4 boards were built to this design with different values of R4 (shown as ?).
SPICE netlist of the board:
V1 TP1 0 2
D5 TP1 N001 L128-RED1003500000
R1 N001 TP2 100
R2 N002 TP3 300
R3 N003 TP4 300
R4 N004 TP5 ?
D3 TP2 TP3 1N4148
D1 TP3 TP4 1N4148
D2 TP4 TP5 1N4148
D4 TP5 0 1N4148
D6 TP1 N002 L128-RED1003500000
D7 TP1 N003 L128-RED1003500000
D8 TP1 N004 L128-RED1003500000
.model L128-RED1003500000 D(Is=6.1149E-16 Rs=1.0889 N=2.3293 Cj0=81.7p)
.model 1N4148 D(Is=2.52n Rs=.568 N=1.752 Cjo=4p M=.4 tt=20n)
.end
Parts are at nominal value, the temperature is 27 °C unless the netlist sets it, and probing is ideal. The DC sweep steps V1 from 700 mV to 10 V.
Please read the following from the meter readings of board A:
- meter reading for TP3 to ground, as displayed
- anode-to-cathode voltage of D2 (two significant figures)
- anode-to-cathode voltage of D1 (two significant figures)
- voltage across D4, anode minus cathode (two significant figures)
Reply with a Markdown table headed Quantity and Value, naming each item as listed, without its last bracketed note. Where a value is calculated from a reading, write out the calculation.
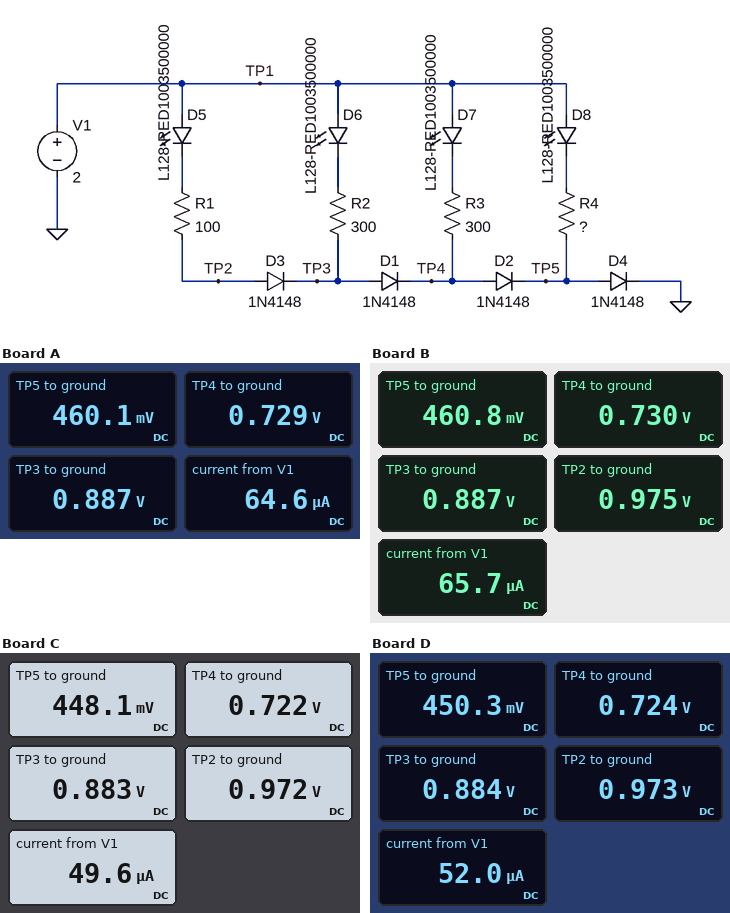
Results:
| Quantity | Value |
|---|---|
| meter reading for TP3 to ground, as displayed | 0.887 V |
| anode-to-cathode voltage of D2 | 729 mV - 460.1 mV = 270 mV |
| anode-to-cathode voltage of D1 | 887 mV - 729 mV = 160 mV |
| voltage across D4, anode minus cathode | 460.1 mV = 460 mV |
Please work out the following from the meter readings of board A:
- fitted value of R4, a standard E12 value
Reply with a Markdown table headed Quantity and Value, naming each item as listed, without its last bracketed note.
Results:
| Quantity | Value |
|---|---|
| fitted value of R4, a standard E12 value | 180 Ω |
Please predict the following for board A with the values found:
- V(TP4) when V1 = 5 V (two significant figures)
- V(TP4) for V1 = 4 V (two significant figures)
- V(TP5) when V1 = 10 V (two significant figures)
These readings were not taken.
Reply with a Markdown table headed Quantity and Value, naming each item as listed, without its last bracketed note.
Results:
| Quantity | Value |
|---|---|
| V(TP4) when V1 = 5 V | 1.5 V |
| V(TP4) for V1 = 4 V | 1.4 V |
| V(TP5) when V1 = 10 V | 880 mV |
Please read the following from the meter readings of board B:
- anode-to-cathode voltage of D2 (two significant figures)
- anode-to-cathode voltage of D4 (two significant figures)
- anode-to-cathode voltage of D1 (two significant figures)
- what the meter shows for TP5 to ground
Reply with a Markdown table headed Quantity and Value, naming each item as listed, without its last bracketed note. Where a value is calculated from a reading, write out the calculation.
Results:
| Quantity | Value |
|---|---|
| anode-to-cathode voltage of D2 | 730 mV - 460.8 mV = 270 mV |
| anode-to-cathode voltage of D4 | 460.8 mV = 460 mV |
| anode-to-cathode voltage of D1 | 887 mV - 730 mV = 160 mV |
| what the meter shows for TP5 to ground | 460.8 mV |
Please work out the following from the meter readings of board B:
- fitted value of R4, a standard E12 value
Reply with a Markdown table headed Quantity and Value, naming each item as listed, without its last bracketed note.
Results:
| Quantity | Value |
|---|---|
| fitted value of R4, a standard E12 value | 150 Ω |
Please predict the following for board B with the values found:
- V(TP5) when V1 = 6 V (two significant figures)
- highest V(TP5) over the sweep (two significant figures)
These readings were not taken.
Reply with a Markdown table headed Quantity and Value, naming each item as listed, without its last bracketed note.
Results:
| Quantity | Value |
|---|---|
| V(TP5) when V1 = 6 V | 790 mV |
| highest V(TP5) over the sweep | 880 mV |
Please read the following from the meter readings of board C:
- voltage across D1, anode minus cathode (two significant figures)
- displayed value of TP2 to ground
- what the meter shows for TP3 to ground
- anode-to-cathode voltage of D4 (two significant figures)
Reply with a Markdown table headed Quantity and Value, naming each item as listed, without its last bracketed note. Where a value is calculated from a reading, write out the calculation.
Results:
| Quantity | Value |
|---|---|
| voltage across D1, anode minus cathode | 883 mV - 722 mV = 160 mV |
| displayed value of TP2 to ground | 0.972 V |
| what the meter shows for TP3 to ground | 0.883 V |
| anode-to-cathode voltage of D4 | 448.1 mV = 450 mV |
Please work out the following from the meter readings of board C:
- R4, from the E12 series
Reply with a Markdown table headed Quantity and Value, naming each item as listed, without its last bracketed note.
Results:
| Quantity | Value |
|---|---|
| R4, from the E12 series | 820 Ω |
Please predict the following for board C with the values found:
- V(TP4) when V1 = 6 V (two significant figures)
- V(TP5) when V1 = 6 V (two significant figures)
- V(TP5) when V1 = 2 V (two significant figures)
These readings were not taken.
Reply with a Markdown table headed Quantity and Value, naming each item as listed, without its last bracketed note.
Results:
| Quantity | Value |
|---|---|
| V(TP4) when V1 = 6 V | 1.5 V |
| V(TP5) when V1 = 6 V | 760 mV |
| V(TP5) when V1 = 2 V | 450 mV |
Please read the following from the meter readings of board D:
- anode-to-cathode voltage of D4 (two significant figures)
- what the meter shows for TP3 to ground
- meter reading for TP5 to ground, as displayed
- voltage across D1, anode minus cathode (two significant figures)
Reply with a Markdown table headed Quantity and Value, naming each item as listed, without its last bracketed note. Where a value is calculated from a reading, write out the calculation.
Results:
| Quantity | Value |
|---|---|
| anode-to-cathode voltage of D4 | 450.3 mV = 450 mV |
| what the meter shows for TP3 to ground | 0.884 V |
| meter reading for TP5 to ground, as displayed | 450.3 mV |
| voltage across D1, anode minus cathode | 884 mV - 724 mV = 160 mV |
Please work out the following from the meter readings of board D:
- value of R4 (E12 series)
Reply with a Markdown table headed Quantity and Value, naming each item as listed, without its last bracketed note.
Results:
| Quantity | Value |
|---|---|
| value of R4 | 680 Ω |
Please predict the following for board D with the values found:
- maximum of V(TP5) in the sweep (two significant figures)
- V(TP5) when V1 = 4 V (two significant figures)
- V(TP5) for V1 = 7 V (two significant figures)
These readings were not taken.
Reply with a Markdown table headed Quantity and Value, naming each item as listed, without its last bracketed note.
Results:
| Quantity | Value |
|---|---|
| maximum of V(TP5) in the sweep | 850 mV |
| V(TP5) when V1 = 4 V | 670 mV |
| V(TP5) for V1 = 7 V | 790 mV |
